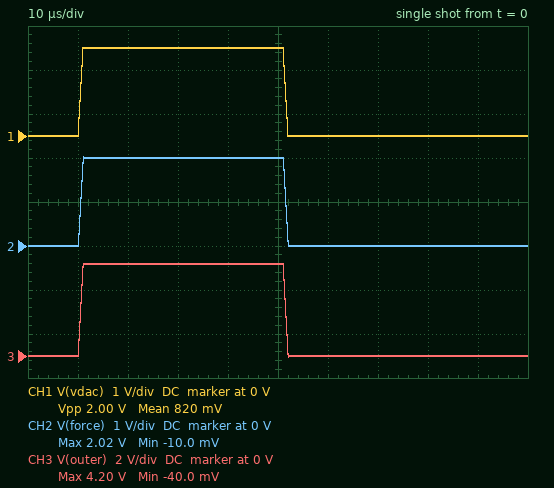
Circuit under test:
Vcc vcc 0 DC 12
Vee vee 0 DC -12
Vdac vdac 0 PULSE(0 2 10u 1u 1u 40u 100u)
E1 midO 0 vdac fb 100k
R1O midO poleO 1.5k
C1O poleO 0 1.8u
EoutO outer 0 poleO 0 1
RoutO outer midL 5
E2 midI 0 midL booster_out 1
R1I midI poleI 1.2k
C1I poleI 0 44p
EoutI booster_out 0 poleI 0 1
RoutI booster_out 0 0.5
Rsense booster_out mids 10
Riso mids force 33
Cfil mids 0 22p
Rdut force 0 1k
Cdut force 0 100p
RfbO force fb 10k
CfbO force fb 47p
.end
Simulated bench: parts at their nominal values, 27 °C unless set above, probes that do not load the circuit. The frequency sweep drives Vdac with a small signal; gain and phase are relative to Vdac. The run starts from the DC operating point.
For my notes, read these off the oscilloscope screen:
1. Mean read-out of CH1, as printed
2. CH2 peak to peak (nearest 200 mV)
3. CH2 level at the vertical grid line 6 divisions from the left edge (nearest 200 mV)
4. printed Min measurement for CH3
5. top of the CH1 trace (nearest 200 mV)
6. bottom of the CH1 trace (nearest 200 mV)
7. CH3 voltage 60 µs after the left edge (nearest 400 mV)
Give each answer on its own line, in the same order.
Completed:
820 mV
2.0 V
0 V
-40.0 mV
2.0 V
0 V
0 V
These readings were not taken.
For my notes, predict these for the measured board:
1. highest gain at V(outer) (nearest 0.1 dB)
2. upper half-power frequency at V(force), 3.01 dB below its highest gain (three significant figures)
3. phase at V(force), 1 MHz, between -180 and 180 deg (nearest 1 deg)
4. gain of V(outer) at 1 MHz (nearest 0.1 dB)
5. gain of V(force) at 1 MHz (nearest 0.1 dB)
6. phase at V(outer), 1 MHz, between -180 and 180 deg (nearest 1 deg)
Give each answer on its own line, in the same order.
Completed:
6.8 dB
4.27 MHz
-21 deg
6.5 dB
0 dB
-10 deg
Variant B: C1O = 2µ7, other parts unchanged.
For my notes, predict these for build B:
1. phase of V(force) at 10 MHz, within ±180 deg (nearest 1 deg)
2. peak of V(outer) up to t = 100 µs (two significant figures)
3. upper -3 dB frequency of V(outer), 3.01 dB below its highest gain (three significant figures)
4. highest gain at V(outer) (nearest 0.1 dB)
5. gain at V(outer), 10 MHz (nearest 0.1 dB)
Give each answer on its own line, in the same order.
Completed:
-163 deg
4.2 V
3.16 MHz
6.4 dB
-7.3 dB
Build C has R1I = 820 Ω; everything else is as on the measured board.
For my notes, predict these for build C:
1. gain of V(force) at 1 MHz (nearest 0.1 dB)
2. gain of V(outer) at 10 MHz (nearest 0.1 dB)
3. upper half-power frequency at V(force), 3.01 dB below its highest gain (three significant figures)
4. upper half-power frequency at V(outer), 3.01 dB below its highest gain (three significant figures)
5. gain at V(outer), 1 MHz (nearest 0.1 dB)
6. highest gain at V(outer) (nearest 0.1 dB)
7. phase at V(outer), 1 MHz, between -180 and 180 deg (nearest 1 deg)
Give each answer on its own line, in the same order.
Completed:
-0.1 dB
-3.1 dB
4.22 MHz
4.96 MHz
6.3 dB
6.4 dB
-12 deg
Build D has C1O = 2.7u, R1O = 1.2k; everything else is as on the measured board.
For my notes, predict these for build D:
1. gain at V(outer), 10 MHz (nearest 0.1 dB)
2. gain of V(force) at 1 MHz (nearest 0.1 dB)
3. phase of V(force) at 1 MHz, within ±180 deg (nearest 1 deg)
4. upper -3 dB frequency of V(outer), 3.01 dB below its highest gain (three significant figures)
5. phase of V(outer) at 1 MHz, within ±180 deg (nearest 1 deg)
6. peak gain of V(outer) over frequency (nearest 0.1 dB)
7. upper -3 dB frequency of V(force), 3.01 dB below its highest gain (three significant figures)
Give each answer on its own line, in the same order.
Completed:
-5.1 dB
-0.1 dB
-25 deg
4.28 MHz
-14 deg
6.4 dB
3.53 MHz
